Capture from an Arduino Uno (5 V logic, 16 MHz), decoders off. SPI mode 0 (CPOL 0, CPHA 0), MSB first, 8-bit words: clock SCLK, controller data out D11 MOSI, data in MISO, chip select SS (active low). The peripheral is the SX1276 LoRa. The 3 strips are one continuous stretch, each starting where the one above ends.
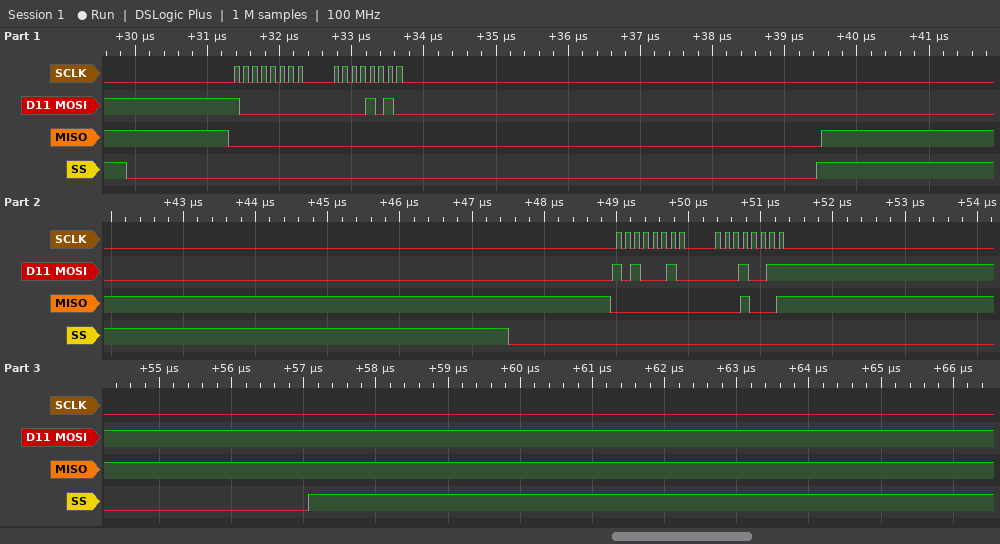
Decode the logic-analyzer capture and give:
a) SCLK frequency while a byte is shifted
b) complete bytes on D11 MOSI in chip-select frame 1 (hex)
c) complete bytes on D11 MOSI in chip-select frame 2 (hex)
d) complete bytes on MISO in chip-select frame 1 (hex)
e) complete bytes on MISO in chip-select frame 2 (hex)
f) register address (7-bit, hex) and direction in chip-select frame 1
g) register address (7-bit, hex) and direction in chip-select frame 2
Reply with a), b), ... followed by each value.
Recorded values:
a) 8 MHz
b) 80 0A
c) A2 13
d) 00 00
e) 00 11
f) 0x00 write
g) 0x22 write
